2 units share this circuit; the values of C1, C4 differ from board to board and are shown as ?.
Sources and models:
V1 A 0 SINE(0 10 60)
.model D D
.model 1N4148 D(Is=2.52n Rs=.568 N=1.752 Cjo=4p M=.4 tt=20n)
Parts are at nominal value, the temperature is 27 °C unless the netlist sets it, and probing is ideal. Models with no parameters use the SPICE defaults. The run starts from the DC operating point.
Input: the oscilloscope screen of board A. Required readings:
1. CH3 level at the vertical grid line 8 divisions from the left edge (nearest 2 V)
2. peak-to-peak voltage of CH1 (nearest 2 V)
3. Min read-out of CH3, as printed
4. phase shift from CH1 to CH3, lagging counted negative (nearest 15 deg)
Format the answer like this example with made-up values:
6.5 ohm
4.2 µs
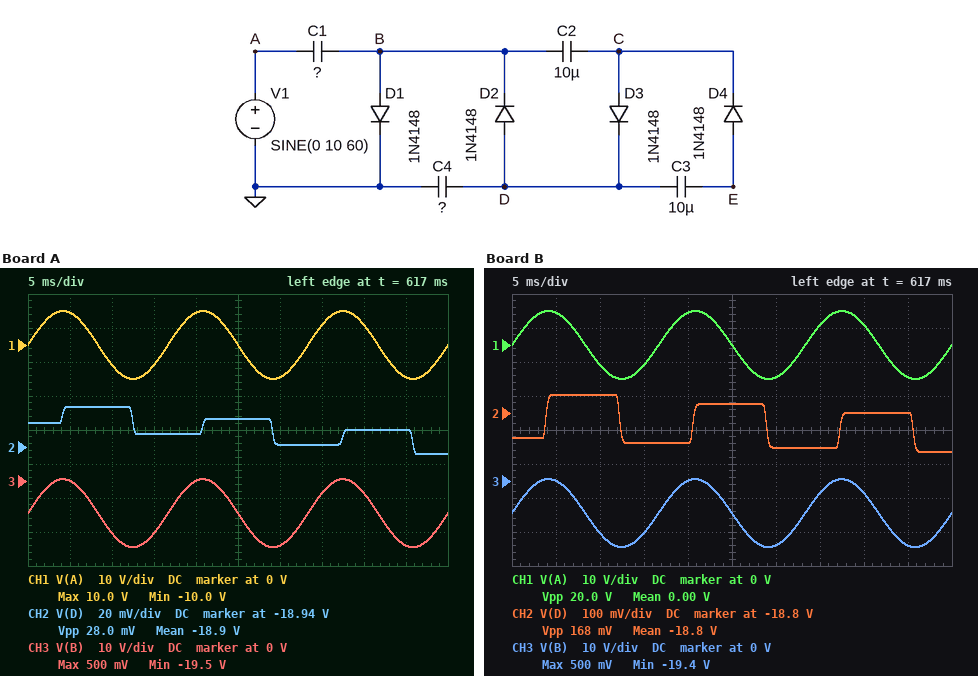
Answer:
-4 V
20 V
-19.5 V
0 deg
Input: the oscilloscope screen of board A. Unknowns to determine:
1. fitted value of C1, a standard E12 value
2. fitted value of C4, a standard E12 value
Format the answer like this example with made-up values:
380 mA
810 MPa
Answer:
12 µF
15 µF
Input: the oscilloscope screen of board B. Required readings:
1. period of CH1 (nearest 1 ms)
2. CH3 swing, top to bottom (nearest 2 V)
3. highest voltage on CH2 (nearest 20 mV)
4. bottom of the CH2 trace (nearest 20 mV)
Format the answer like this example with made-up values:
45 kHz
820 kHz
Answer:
17 ms
20 V
-18.74 V
-18.92 V
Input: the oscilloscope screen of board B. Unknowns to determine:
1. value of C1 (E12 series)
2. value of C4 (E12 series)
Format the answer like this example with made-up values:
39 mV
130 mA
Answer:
8.2 µF
4.7 µF
